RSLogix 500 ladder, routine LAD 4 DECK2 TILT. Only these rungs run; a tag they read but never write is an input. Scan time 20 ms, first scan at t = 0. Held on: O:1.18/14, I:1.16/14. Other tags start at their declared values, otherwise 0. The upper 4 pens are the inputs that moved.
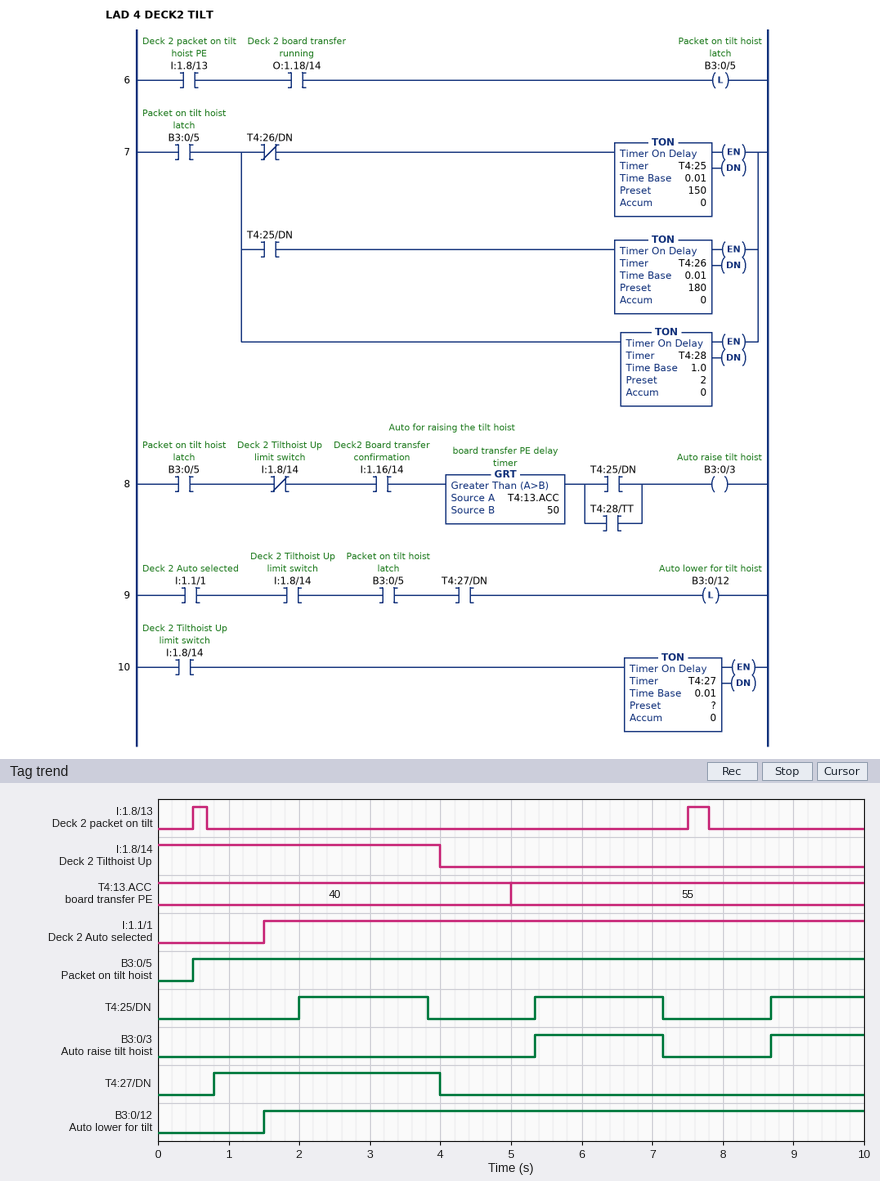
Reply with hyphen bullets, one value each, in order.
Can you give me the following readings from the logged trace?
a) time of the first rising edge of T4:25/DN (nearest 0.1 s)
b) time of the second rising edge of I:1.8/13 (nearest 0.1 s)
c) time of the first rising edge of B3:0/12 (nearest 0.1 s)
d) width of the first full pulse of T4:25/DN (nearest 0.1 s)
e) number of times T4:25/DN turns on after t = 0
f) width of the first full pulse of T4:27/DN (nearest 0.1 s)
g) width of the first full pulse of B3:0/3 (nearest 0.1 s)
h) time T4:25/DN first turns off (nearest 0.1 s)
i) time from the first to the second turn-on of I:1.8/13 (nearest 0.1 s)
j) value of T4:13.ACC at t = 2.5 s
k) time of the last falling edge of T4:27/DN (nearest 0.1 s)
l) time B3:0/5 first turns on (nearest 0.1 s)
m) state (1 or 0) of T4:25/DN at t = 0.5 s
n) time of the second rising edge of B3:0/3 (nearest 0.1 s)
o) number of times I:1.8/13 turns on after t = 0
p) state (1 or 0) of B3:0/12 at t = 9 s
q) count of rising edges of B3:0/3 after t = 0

- 2.0 s
- 7.5 s
- 1.5 s
- 1.8 s
- 3
- 3.2 s
- 1.8 s
- 3.8 s
- 7.0 s
- 40
- 4.0 s
- 0.5 s
- 0
- 8.7 s
- 2
- 1
- 2
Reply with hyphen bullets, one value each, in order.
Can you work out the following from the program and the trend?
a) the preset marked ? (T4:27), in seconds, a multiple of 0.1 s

- 0.8 s
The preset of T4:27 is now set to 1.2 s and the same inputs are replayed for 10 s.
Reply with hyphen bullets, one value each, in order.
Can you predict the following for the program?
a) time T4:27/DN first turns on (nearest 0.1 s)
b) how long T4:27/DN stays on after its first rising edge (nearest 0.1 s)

- 1.2 s
- 2.8 s
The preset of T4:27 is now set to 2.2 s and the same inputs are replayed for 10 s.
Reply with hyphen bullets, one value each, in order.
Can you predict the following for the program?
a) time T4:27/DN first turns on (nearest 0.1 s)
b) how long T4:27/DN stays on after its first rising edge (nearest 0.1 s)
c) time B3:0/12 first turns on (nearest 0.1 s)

- 2.2 s
- 1.8 s
- 2.2 s
